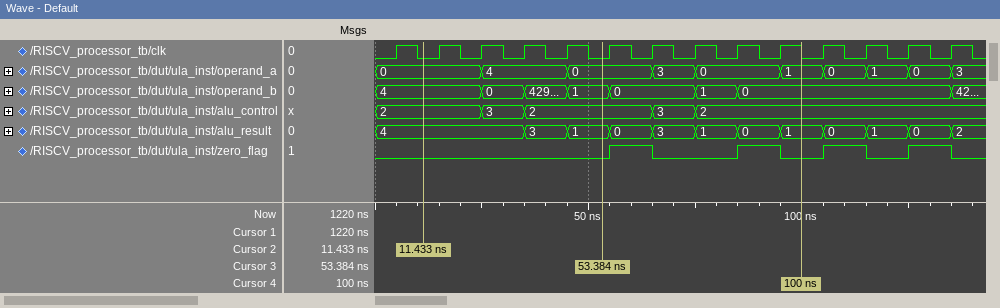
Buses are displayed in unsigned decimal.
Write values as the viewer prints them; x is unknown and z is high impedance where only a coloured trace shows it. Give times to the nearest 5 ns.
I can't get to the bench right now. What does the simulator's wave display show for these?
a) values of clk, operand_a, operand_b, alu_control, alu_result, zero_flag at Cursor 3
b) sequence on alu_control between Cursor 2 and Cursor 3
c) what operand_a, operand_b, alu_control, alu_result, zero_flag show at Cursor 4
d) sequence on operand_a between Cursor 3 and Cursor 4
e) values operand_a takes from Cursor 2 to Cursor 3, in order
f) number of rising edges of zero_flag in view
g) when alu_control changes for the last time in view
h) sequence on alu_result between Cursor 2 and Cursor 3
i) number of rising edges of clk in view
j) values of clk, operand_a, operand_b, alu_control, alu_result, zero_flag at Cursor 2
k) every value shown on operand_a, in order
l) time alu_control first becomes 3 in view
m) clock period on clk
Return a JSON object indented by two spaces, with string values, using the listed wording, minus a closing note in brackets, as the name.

{
  "values of clk, operand_a, operand_b, alu_control, alu_result, zero_flag at Cursor 3": "clk=0, operand_a=0, operand_b=1, alu_control=2, alu_result=1, zero_flag=0",
  "sequence on alu_control between Cursor 2 and Cursor 3": "2, 3, 2",
  "what operand_a, operand_b, alu_control, alu_result, zero_flag show at Cursor 4": "operand_a=1, operand_b=0, alu_control=2, alu_result=1, zero_flag=0",
  "sequence on operand_a between Cursor 3 and Cursor 4": "0, 3, 0, 1",
  "values operand_a takes from Cursor 2 to Cursor 3, in order": "0, 4, 0",
  "number of rising edges of zero_flag in view": "4",
  "when alu_control changes for the last time in view": "75 ns",
  "sequence on alu_result between Cursor 2 and Cursor 3": "4, 3, 1",
  "number of rising edges of clk in view": "14",
  "values of clk, operand_a, operand_b, alu_control, alu_result, zero_flag at Cursor 2": "clk=0, operand_a=0, operand_b=4, alu_control=2, alu_result=4, zero_flag=0",
  "every value shown on operand_a, in order": "0, 4, 0, 3, 0, 1, 0, 1, 0, 3",
  "time alu_control first becomes 3 in view": "25 ns",
  "clock period on clk": "10 ns"
}
